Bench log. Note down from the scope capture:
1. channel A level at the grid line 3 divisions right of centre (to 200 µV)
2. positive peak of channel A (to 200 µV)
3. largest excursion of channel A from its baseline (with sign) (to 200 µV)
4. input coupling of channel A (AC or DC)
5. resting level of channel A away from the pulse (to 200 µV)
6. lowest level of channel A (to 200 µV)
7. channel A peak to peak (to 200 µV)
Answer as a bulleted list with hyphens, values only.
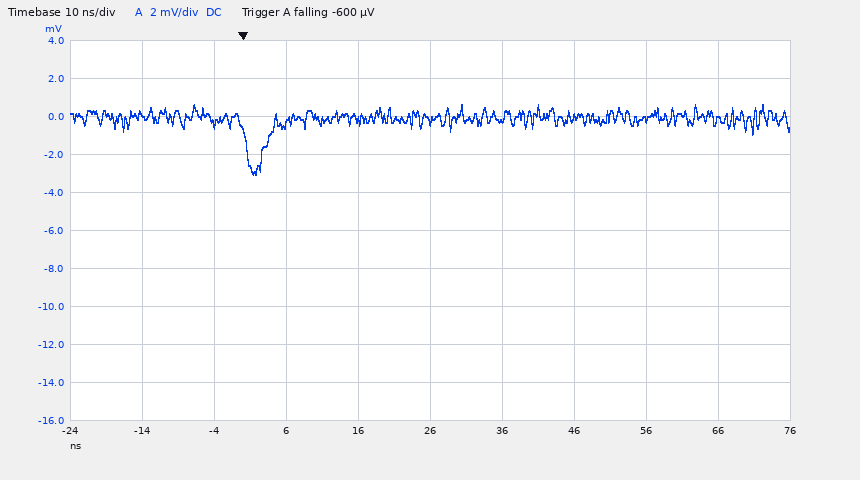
- -200 µV
- 600 µV
- -3.0 mV
- DC
- 0.0 mV
- -3.0 mV
- 3.6 mV
